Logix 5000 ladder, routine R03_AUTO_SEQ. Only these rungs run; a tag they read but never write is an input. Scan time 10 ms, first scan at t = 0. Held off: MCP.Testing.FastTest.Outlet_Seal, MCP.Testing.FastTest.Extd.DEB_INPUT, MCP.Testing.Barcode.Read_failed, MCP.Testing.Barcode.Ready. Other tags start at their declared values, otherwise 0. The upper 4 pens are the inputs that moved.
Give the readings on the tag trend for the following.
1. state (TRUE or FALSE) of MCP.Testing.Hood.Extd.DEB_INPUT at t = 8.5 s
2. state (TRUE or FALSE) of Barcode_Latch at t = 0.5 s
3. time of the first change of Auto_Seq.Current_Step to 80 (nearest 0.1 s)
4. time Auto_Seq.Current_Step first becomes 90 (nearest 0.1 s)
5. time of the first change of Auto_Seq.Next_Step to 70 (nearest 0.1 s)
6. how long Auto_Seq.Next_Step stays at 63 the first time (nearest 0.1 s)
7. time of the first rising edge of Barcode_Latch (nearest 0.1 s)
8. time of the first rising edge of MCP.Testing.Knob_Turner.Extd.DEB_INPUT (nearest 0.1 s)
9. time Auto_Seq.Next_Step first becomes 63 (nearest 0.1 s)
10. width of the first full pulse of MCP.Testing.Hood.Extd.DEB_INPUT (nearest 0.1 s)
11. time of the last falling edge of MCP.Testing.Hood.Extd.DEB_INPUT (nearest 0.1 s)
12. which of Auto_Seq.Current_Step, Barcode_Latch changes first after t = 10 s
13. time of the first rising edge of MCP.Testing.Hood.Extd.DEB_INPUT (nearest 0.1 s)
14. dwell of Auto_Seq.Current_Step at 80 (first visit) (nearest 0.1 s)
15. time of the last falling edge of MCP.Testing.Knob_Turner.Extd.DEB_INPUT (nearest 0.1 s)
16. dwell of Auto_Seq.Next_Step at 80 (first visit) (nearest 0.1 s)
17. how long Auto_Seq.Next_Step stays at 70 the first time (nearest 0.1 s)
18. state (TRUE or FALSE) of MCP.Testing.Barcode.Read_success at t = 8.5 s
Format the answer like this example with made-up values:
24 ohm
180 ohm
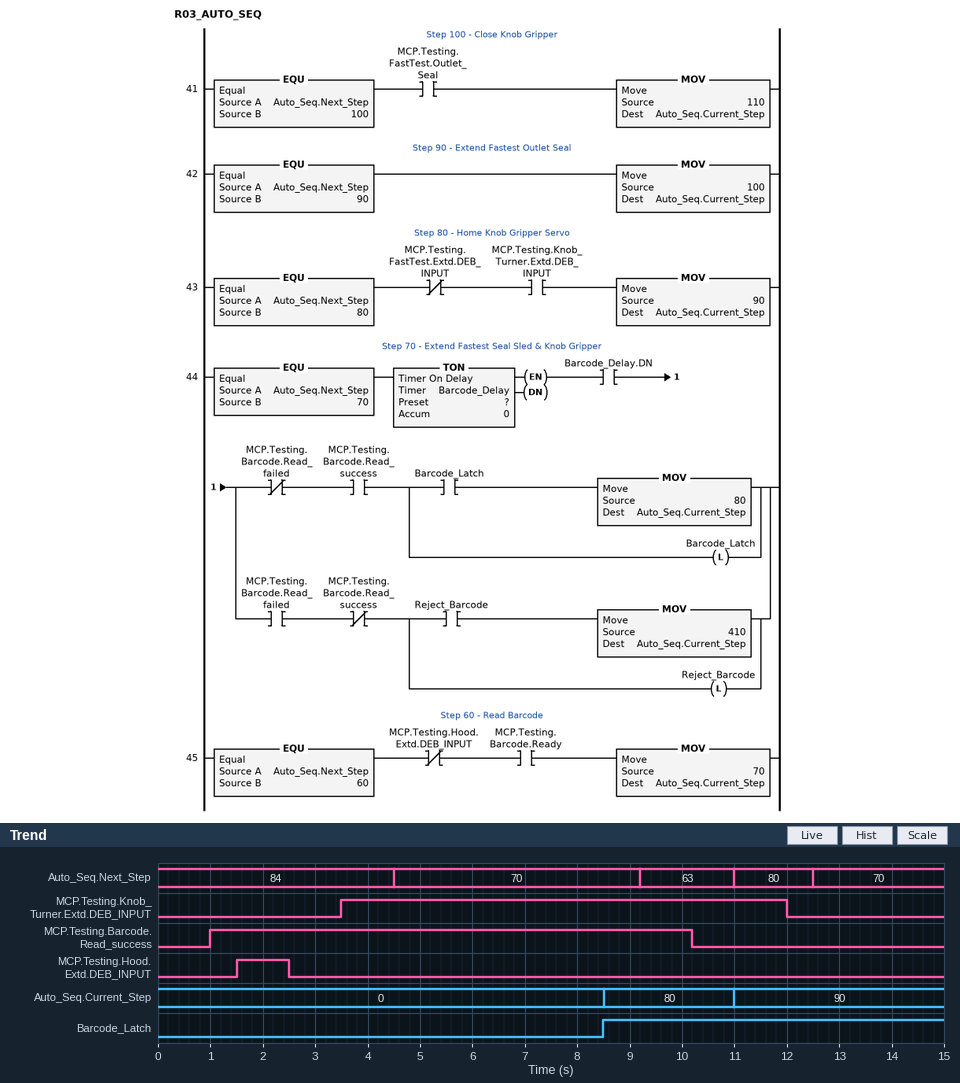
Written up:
FALSE
FALSE
8.5 s
11.0 s
4.5 s
1.8 s
8.5 s
3.5 s
9.2 s
1.0 s
2.5 s
Auto_Seq.Current_Step
1.5 s
2.5 s
12.0 s
1.5 s
4.7 s
TRUE
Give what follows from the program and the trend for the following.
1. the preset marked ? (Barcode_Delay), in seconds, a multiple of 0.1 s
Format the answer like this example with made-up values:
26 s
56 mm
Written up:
4.0 s
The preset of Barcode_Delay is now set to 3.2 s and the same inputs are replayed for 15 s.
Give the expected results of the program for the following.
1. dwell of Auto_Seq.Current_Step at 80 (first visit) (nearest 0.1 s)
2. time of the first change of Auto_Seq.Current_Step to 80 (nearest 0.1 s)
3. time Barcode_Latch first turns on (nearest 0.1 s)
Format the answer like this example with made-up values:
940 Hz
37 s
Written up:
3.3 s
7.7 s
7.7 s
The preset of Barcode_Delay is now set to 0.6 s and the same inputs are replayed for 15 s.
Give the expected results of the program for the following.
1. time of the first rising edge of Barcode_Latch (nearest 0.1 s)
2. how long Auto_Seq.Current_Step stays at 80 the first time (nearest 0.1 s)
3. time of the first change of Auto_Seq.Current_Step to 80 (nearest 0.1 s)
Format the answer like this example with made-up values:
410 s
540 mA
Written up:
5.1 s
5.9 s
5.1 s
